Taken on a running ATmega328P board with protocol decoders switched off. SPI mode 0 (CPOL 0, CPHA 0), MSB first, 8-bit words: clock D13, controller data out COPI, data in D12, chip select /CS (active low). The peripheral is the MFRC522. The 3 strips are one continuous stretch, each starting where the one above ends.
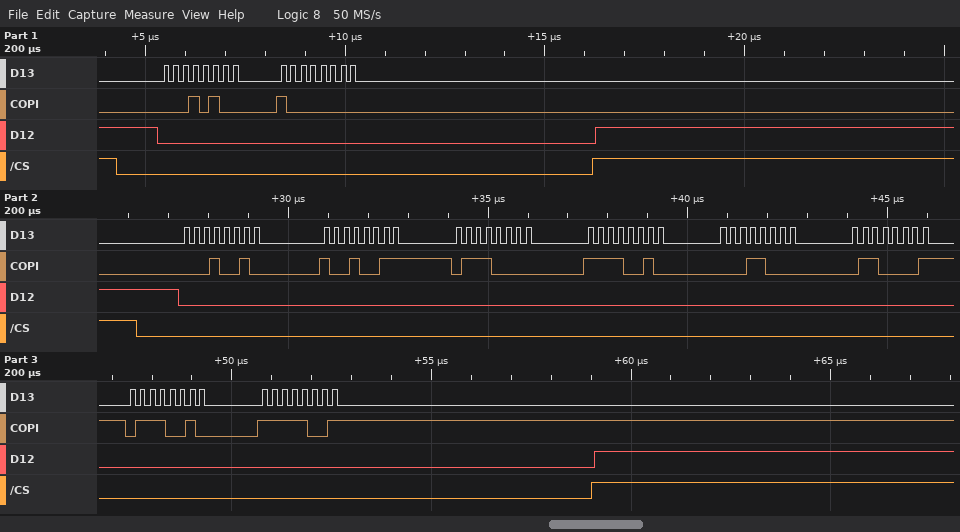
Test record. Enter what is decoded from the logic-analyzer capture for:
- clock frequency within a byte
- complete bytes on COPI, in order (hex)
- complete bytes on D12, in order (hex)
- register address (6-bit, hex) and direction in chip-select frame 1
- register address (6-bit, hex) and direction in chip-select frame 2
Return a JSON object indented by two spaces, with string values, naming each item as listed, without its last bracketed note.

{
  "clock frequency within a byte": "4 MHz",
  "complete bytes on COPI, in order": "14 80 12 93 70 F2 18 61 72 F9",
  "complete bytes on D12, in order": "00 00 00 00 00 00 00 00 00 00",
  "register address (6-bit, hex) and direction in chip-select frame 1": "0x0A write",
  "register address (6-bit, hex) and direction in chip-select frame 2": "0x09 write"
}
